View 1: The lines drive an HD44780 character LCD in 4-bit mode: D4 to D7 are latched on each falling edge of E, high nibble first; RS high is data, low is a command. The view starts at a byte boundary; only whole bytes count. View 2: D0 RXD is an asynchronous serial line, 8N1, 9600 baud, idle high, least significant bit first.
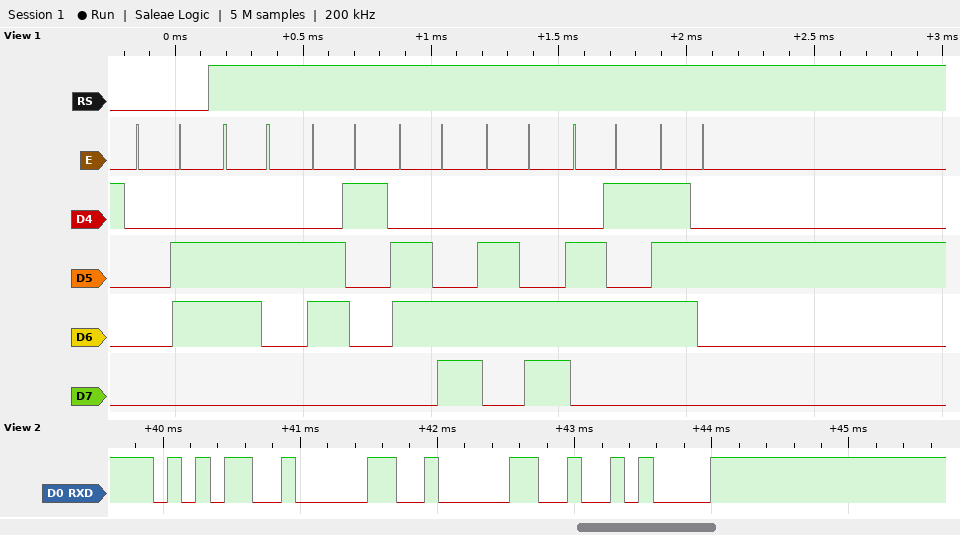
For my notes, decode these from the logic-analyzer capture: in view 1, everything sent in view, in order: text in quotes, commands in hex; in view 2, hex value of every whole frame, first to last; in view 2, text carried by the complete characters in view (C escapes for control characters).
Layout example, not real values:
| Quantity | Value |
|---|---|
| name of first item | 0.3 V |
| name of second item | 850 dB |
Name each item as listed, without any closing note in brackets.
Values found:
| Quantity | Value |
|---|---|
| in view 1, everything sent in view, in order: text in quotes, commands in hex | 0x06 "baller" |
| in view 2, hex value of every whole frame, first to last | 35 30 30 0A |
| in view 2, text carried by the complete characters in view | "500\n" |
